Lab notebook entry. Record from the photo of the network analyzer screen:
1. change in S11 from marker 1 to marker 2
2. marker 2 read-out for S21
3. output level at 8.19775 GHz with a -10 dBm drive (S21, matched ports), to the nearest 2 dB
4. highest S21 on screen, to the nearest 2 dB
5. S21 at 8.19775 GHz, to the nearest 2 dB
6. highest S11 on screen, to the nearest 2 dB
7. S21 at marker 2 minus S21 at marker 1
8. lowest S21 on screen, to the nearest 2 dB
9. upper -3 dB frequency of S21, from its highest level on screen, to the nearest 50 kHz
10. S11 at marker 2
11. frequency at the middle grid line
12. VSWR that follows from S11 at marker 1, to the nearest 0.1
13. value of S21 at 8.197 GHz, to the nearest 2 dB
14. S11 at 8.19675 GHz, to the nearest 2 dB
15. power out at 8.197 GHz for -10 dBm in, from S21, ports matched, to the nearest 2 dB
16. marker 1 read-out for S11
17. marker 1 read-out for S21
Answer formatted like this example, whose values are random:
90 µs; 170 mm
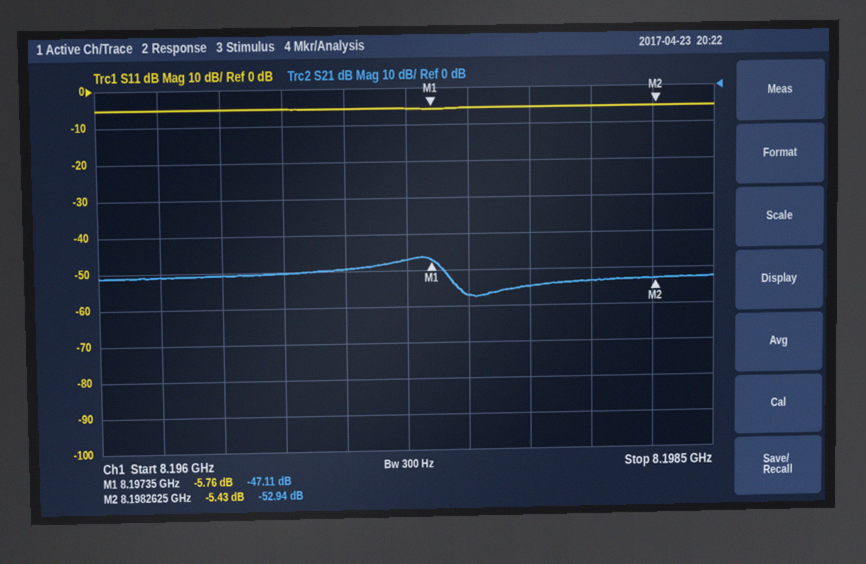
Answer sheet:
0.33 dB; -52.94 dB; -64 dBm; -46 dB; -54 dB; -6 dB; -5.83 dB; -58 dB; 8.19740 GHz; -5.43 dB; 8.19725 GHz; 3.1; -50 dB; -6 dB; -60 dBm; -5.76 dB; -47.11 dB
